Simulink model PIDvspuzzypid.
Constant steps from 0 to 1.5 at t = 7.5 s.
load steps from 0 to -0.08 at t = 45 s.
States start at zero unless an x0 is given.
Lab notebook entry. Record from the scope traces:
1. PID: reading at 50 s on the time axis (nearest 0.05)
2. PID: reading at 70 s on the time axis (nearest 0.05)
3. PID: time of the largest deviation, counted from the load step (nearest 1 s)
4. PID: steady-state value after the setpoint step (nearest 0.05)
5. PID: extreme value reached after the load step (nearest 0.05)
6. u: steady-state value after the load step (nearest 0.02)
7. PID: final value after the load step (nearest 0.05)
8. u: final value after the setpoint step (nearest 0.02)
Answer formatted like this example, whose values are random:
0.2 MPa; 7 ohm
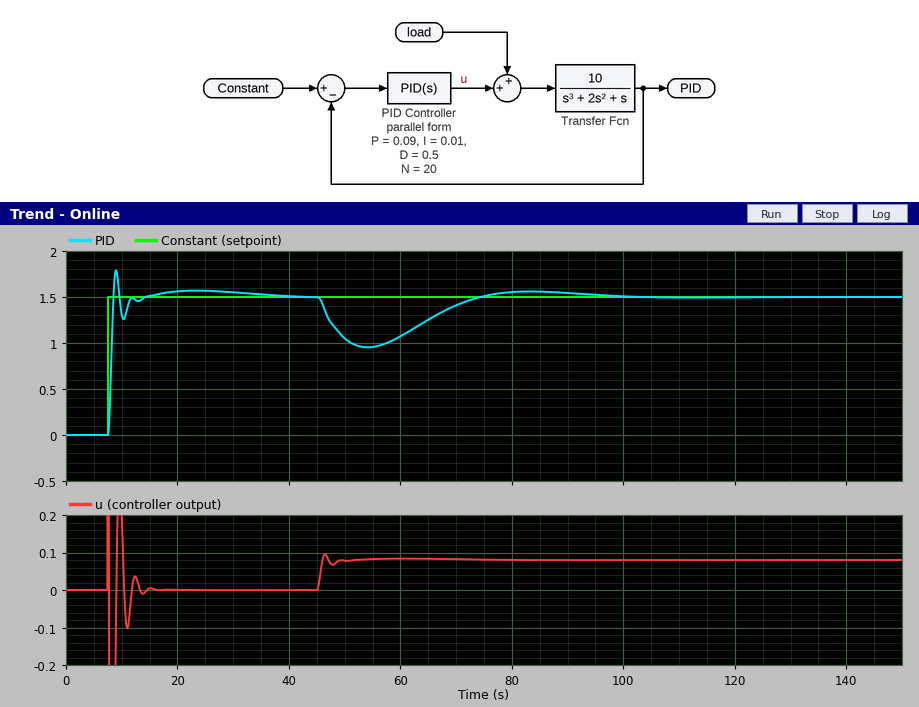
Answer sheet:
1.05; 1.40; 9 s; 1.50; 0.95; 0.08; 1.50; 0.00
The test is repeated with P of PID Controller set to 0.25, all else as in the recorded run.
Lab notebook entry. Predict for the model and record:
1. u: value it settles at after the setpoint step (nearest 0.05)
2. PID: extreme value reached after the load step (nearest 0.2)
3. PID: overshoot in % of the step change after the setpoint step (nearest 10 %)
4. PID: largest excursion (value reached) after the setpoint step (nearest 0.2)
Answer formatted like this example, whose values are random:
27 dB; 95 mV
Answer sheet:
0.00; 1.2; 40 %; 2.0
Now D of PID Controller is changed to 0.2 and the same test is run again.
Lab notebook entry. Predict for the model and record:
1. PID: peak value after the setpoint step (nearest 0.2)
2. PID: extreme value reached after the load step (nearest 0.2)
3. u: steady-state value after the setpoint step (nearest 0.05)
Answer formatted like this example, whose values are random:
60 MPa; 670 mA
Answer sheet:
1.6; 0.8; 0.00
